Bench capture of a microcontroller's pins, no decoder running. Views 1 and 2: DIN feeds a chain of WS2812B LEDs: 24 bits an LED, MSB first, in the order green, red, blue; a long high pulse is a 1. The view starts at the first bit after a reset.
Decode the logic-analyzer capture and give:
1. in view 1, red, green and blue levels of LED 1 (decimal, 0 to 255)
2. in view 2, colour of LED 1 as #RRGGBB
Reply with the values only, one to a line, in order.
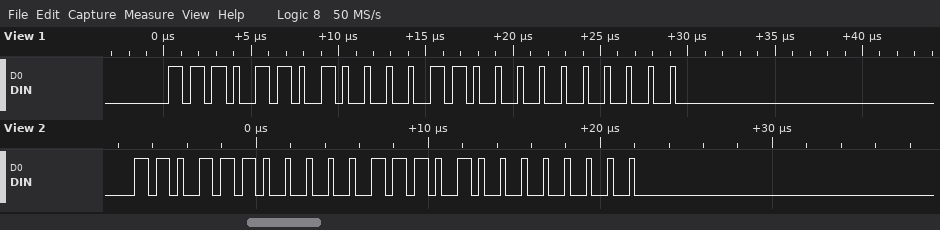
12, 237, 0
#1DDC00
